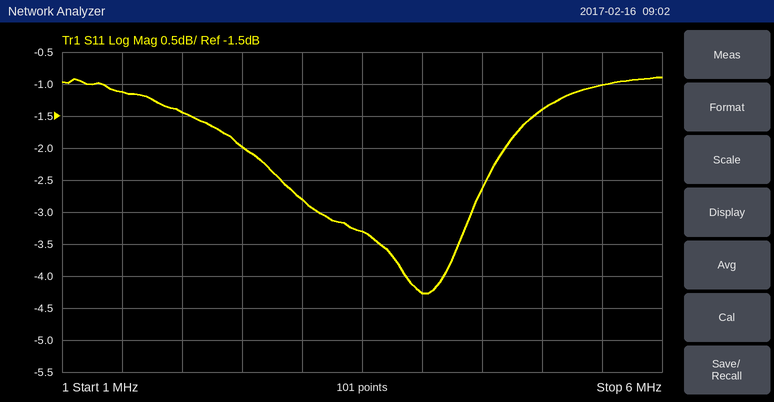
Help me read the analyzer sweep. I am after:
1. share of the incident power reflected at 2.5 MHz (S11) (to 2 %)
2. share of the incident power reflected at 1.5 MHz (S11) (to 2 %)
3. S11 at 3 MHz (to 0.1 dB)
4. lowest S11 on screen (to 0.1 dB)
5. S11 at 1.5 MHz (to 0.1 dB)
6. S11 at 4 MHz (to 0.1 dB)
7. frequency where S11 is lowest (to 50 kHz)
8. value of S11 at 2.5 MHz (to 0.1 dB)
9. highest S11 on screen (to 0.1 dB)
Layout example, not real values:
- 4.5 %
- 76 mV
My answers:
- 64 %
- 78 %
- -2.8 dB
- -4.3 dB
- -1.1 dB
- -4.3 dB
- 4.00 MHz
- -2.0 dB
- -0.9 dB
